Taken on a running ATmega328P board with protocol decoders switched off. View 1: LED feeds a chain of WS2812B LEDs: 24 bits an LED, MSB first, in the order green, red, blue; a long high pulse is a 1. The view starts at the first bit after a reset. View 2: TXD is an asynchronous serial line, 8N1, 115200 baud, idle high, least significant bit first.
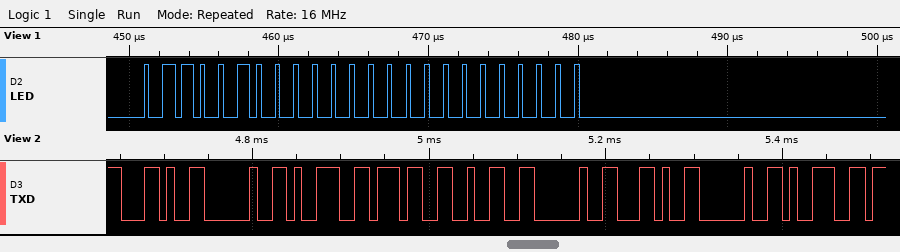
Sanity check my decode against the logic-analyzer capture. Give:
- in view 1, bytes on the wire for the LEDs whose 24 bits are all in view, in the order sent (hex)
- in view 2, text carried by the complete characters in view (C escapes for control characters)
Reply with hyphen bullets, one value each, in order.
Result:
- 64 00 00
- ", 972 , 9"
